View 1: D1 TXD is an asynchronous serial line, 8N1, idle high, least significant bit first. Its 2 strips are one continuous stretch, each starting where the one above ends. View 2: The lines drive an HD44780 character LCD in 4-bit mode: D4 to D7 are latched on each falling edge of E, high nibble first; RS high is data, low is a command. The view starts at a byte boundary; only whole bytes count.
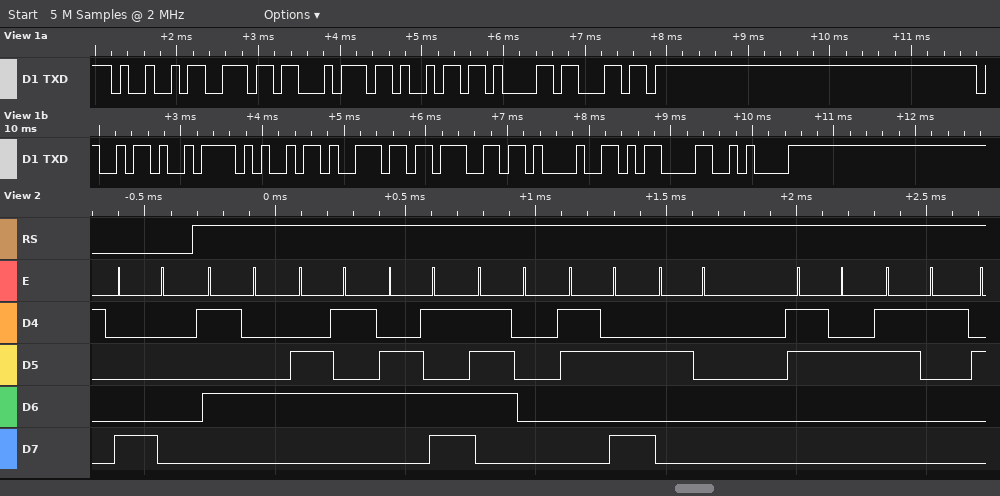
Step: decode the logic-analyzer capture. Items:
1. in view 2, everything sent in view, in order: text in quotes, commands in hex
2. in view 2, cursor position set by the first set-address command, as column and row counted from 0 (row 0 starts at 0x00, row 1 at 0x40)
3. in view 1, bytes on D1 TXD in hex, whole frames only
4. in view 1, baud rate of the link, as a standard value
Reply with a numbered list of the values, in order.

1. 0x80 "Temp: 21"
2. column 0, row 0
3. 0x49 0x6E 0x74 0x69 0x61 0x6C 0x69 0x7A 0x69 0x6E 0x67 0x21 0x0D 0x0A
4. 9600 baud
